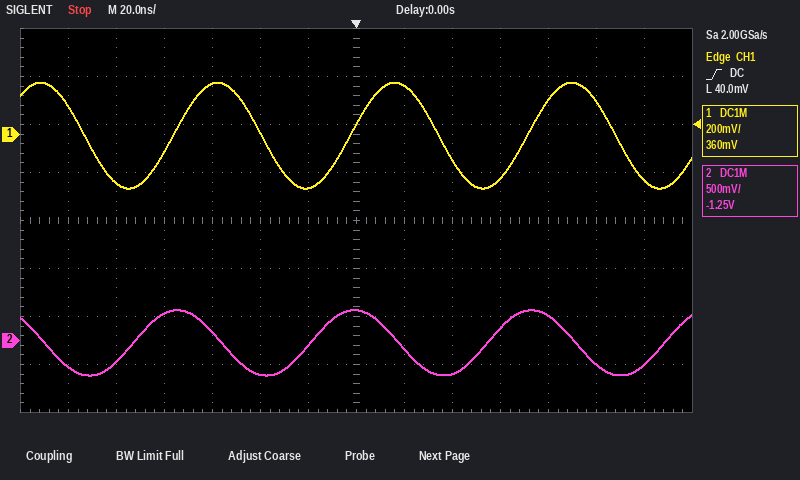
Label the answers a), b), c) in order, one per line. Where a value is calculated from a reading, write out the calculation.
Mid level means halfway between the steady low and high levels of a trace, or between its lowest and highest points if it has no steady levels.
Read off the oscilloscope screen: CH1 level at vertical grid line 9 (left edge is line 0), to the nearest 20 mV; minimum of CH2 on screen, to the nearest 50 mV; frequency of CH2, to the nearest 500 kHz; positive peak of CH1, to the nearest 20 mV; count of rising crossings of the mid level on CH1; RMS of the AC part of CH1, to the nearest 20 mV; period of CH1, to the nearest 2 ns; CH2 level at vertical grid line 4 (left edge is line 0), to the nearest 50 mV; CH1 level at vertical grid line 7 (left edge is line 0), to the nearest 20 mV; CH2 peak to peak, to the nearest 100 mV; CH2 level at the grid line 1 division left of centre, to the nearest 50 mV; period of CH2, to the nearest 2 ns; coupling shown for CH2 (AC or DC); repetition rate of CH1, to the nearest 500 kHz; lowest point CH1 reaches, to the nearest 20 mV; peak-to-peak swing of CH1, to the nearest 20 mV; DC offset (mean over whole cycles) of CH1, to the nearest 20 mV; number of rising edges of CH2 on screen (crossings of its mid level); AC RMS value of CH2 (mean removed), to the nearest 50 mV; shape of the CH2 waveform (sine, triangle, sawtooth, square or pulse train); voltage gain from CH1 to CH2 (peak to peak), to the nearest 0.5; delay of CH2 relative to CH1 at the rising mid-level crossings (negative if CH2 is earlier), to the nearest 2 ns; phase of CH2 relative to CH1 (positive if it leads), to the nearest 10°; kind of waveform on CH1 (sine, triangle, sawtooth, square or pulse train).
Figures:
a) -100 mV
b) -350 mV
c) 1 / 74 ns ≈ 13.5 MHz
d) 220 mV
e) 3
f) 440 mV / (2√2) ≈ 156 mV, so 160 mV to the nearest 20 mV
g) 74 ns
h) 100 mV
i) 40 mV
j) 700 mV
k) -50 mV
l) 74 ns
m) DC
n) 1 / 74 ns ≈ 13.5 MHz
o) -220 mV
p) 220 mV − (-220 mV) = 440 mV
q) (220 mV + (-220 mV)) / 2 ≈ 0 mV
r) 4
s) 700 mV / (2√2) ≈ 247 mV, so 250 mV to the nearest 50 mV
t) sine
u) 700 mV / 440 mV ≈ 1.59, so 1.5 to the nearest 0.5
v) -16 ns
w) −360° × (-16 ns) / 74 ns ≈ +77.8°, so +80° to the nearest 10°
x) sine
